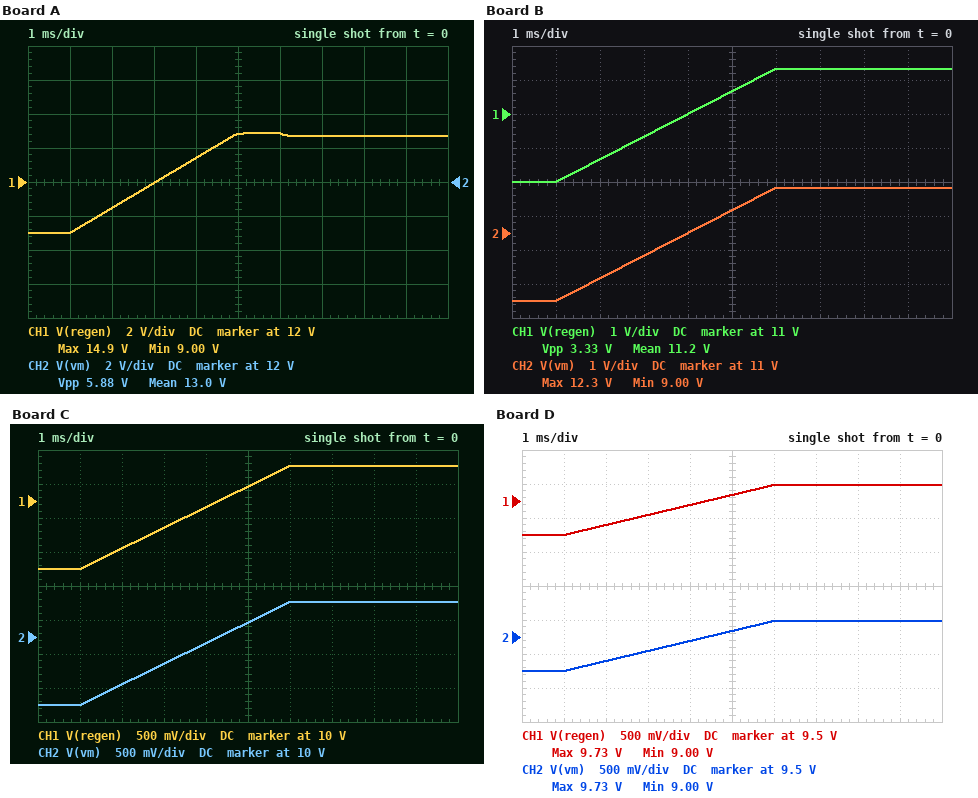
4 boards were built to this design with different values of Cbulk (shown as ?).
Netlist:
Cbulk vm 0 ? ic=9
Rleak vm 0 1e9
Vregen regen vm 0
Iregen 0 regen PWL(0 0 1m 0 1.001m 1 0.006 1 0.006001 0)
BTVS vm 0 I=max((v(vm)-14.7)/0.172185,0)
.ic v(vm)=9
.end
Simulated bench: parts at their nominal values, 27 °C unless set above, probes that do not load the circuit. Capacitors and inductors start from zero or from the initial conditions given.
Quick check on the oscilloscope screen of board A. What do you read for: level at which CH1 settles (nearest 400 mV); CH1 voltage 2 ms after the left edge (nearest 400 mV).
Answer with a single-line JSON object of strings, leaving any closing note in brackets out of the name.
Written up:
{"level at which CH1 settles": "14.8 V", "CH1 voltage 2 ms after the left edge": "10.4 V"}
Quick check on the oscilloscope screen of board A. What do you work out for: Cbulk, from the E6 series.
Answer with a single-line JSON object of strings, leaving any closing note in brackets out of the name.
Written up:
{"Cbulk, from the E6 series": "680 µF"}
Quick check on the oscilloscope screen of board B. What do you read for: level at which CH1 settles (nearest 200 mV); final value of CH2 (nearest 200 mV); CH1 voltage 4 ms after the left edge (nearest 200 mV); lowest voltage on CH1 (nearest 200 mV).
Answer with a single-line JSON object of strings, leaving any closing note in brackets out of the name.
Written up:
{"level at which CH1 settles": "12.4 V", "final value of CH2": "12.4 V", "CH1 voltage 4 ms after the left edge": "11.0 V", "lowest voltage on CH1": "9.0 V"}
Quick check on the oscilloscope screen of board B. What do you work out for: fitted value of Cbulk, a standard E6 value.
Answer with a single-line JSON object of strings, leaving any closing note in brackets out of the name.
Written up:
{"fitted value of Cbulk, a standard E6 value": "1.5 mF"}
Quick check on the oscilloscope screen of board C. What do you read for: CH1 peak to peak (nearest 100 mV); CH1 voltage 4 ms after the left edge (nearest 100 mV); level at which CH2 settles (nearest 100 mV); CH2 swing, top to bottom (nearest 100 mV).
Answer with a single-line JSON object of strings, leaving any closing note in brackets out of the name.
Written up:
{"CH1 peak to peak": "1.5 V", "CH1 voltage 4 ms after the left edge": "9.9 V", "level at which CH2 settles": "10.5 V", "CH2 swing, top to bottom": "1.5 V"}
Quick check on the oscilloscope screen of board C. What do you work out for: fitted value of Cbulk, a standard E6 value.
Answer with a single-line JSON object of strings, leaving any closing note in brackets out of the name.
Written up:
{"fitted value of Cbulk, a standard E6 value": "3.3 mF"}
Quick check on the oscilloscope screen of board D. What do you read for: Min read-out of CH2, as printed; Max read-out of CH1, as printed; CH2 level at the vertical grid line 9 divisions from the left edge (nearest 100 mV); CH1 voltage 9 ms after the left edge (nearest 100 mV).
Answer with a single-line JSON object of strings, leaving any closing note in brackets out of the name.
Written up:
{"Min read-out of CH2, as printed": "9.00 V", "Max read-out of CH1, as printed": "9.73 V", "CH2 level at the vertical grid line 9 divisions from the left edge": "9.7 V", "CH1 voltage 9 ms after the left edge": "9.7 V"}
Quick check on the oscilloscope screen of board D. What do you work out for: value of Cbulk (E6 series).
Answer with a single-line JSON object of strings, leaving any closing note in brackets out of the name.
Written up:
{"value of Cbulk": "6.8 mF"}
